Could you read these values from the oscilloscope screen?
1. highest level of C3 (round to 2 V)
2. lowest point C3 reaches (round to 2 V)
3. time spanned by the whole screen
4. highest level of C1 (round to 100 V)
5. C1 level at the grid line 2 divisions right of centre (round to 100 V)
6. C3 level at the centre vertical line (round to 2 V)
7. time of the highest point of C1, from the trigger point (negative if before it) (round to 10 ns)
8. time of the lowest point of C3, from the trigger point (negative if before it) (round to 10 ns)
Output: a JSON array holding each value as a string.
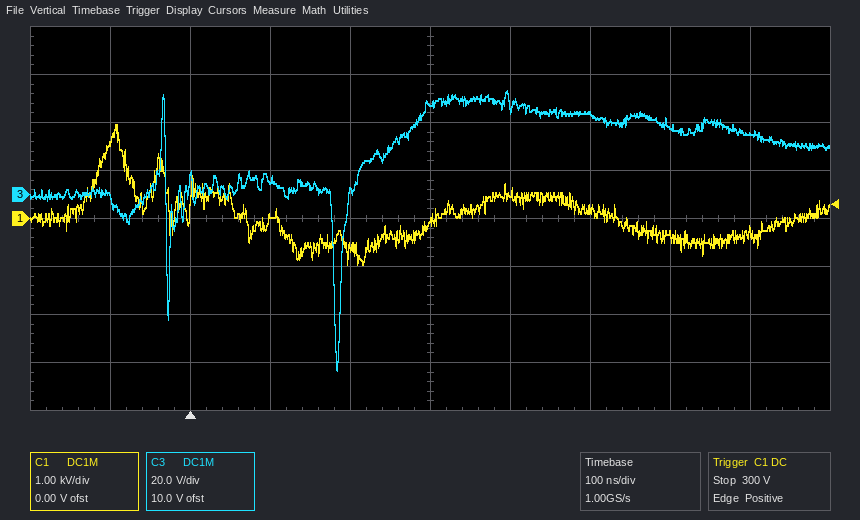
["44 V", "-74 V", "1 µs", "2.0 kV", "200 V", "38 V", "-90 ns", "+180 ns"]
